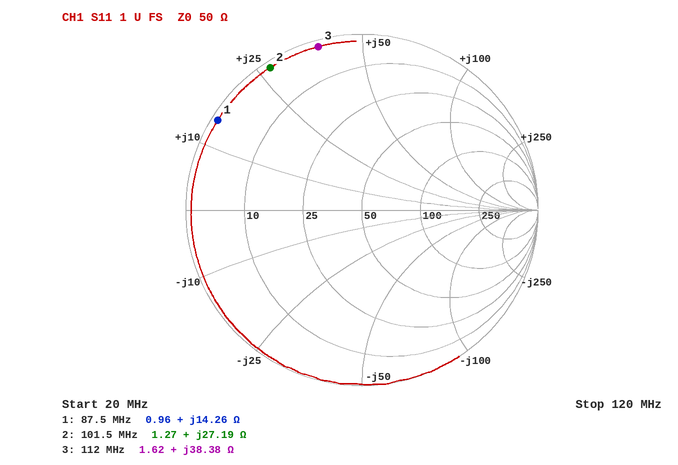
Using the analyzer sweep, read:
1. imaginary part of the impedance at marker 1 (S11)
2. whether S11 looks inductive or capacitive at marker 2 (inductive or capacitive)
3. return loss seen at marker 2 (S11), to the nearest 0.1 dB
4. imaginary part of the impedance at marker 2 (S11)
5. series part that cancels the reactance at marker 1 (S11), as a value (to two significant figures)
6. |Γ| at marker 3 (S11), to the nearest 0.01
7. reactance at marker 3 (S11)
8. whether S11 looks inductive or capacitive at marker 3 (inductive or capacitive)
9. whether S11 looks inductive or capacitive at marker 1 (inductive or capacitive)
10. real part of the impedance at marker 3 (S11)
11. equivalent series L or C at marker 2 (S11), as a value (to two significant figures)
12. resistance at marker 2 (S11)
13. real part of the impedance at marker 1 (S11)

+14.26 Ω
inductive
0.3 dB
+27.19 Ω
130 pF
0.96
+38.38 Ω
inductive
inductive
1.62 Ω
43 nH
1.27 Ω
0.96 Ω
